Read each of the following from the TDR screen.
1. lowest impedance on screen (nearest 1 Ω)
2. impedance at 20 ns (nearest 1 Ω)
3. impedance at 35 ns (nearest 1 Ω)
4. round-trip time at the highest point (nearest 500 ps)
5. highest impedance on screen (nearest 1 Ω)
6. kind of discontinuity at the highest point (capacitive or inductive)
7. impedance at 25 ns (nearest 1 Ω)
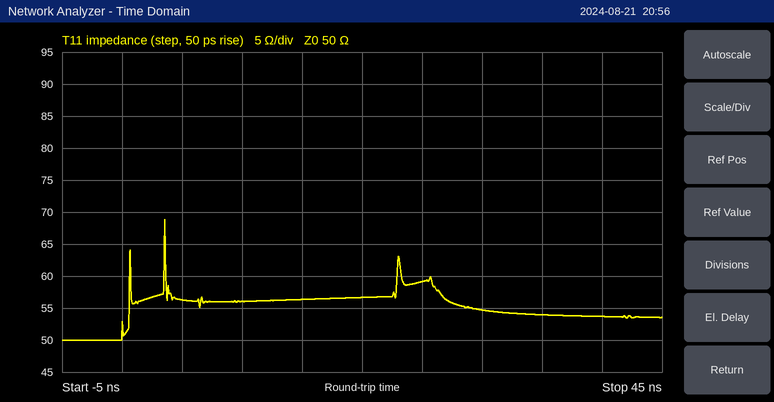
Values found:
50 Ω
57 Ω
54 Ω
3.5 ns
69 Ω
inductive
59 Ω
